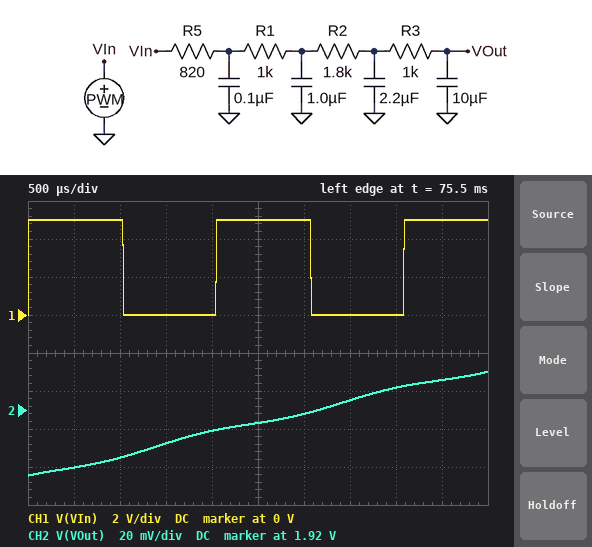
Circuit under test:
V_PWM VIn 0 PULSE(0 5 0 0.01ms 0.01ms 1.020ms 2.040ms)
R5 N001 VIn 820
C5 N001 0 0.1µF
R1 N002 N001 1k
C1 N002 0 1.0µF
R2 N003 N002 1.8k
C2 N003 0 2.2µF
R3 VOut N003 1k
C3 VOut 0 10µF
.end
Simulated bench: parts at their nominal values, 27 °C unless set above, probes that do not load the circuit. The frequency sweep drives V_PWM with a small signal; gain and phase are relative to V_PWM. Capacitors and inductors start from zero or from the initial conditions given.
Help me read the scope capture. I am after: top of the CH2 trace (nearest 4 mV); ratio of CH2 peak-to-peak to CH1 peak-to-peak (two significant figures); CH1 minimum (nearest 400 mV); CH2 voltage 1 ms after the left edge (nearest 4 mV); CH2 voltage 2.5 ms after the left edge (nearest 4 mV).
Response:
1.940 V
0.011
0 V
1.896 V
1.912 V
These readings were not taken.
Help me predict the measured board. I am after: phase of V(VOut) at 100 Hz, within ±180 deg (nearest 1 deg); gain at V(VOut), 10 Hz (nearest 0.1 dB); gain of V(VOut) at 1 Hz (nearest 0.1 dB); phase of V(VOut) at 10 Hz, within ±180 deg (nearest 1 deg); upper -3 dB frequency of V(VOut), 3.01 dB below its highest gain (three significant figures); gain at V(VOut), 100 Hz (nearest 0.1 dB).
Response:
-164 deg
-11.0 dB
-0.5 dB
-83 deg
2.97 Hz
-35.0 dB
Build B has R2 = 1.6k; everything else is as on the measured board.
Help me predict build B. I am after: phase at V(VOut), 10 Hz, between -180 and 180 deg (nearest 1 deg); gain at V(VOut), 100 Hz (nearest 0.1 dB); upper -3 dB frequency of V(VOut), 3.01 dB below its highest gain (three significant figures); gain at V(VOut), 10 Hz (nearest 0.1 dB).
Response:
-82 deg
-34.5 dB
3.11 Hz
-10.6 dB
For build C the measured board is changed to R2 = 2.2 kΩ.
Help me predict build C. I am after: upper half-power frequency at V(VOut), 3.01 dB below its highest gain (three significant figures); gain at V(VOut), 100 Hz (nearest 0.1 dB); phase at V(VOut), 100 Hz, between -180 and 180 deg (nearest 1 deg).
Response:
2.73 Hz
-36.0 dB
-167 deg
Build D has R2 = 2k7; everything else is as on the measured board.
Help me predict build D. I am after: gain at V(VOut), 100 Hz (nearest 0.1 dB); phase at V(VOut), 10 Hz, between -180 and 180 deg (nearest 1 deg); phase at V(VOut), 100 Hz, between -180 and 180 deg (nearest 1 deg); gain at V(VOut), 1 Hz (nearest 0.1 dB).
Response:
-37.1 dB
-86 deg
-170 deg
-0.7 dB
